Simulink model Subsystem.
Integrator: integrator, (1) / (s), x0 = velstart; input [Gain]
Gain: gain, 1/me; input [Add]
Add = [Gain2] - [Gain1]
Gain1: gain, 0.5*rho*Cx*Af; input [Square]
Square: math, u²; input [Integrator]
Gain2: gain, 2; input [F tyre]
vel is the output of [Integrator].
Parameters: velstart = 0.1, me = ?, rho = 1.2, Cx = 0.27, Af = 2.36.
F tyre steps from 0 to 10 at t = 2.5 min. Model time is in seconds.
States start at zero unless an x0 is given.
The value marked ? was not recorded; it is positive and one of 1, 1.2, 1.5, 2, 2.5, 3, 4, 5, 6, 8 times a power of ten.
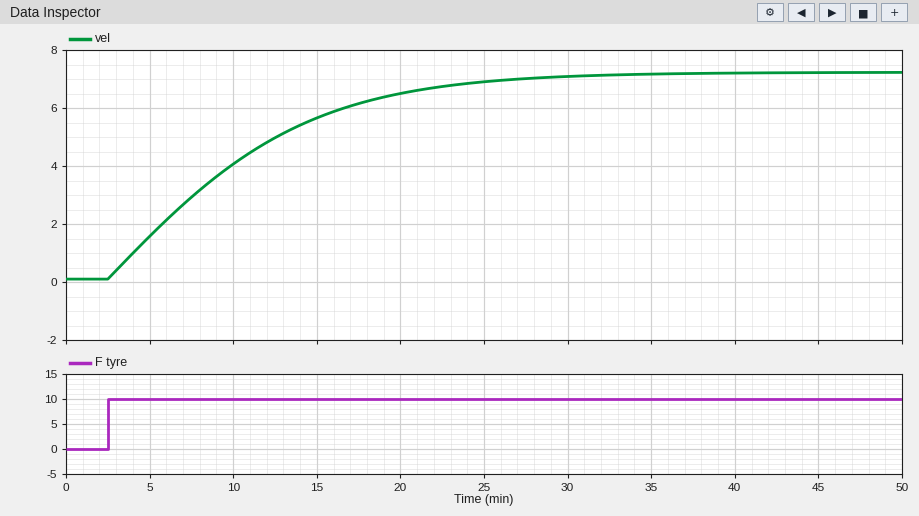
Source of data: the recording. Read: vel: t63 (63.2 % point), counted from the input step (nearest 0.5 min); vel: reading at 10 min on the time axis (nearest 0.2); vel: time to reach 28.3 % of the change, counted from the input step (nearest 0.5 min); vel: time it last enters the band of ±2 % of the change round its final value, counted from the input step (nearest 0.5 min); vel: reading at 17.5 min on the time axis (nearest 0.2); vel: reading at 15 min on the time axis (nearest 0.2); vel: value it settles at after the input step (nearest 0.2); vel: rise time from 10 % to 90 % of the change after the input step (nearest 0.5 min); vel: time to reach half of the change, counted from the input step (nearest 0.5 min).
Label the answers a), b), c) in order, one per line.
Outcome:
a) 9.0 min
b) 4.0
c) 3.5 min
d) 27.5 min
e) 6.2
f) 5.6
g) 7.2
h) 16.5 min
i) 6.5 min
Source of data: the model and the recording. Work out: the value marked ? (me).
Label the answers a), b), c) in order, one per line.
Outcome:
a) 2000
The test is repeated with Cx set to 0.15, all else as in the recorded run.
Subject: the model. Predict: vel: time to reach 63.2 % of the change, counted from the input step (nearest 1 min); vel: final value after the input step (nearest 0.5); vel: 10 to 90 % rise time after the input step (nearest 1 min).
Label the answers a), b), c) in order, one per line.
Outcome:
a) 12 min
b) 9.5
c) 22 min
